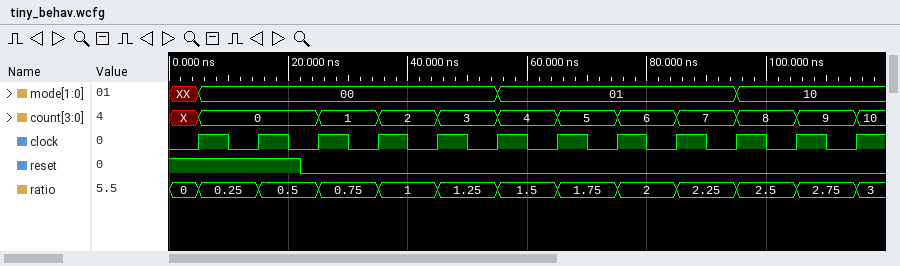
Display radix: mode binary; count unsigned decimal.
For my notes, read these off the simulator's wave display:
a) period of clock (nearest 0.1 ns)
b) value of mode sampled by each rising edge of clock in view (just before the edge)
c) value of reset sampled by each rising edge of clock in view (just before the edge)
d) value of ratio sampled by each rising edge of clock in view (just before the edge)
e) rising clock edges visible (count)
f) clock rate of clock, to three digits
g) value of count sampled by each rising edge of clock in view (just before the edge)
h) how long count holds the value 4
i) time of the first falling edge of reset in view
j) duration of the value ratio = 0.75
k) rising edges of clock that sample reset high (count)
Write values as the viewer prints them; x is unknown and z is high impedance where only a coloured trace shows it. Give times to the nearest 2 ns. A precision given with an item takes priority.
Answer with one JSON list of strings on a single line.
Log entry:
["10 ns", "XX, 00, 00, 00, 00, 00, 01, 01, 01, 01, 10, 10", "1 1 0 0 0 0 0 0 0 0 0 0", "0, 0.25, 0.5, 0.75, 1, 1.25, 1.5, 1.75, 2, 2.25, 2.5, 2.75", "12", "100 MHz", "X, 0, 0, 1, 2, 3, 4, 5, 6, 7, 8, 9", "10 ns", "22 ns", "10 ns", "2"]
